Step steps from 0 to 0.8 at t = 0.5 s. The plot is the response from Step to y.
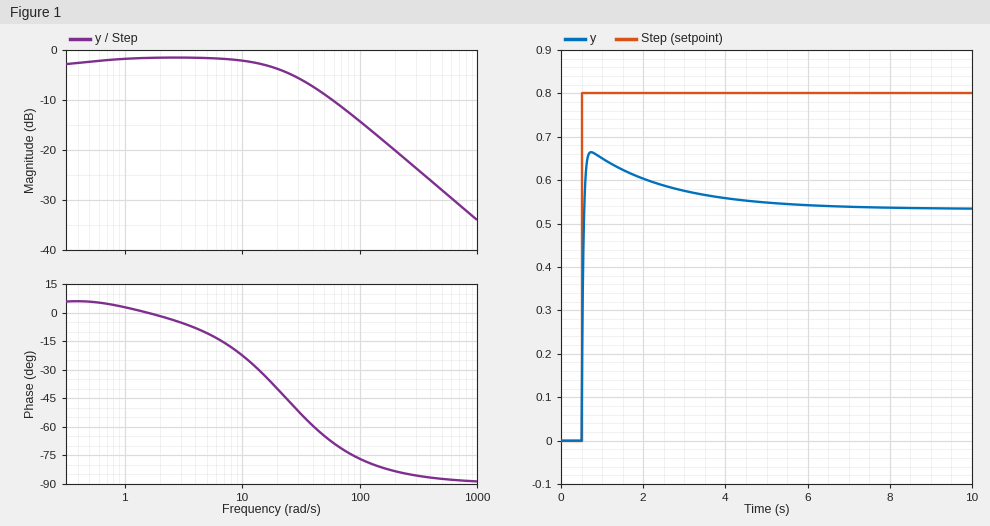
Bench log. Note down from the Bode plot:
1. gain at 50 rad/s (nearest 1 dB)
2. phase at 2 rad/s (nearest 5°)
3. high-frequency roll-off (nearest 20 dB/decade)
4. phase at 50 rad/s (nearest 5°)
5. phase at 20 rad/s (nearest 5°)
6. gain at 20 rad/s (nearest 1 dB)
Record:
-9 dB
0°
-20 dB/decade
-65°
-40°
-4 dB
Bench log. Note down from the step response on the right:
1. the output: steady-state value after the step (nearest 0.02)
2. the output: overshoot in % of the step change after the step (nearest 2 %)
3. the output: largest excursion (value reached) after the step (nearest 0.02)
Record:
0.54
24 %
0.66
